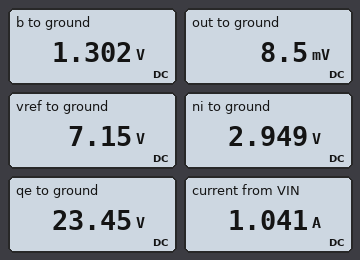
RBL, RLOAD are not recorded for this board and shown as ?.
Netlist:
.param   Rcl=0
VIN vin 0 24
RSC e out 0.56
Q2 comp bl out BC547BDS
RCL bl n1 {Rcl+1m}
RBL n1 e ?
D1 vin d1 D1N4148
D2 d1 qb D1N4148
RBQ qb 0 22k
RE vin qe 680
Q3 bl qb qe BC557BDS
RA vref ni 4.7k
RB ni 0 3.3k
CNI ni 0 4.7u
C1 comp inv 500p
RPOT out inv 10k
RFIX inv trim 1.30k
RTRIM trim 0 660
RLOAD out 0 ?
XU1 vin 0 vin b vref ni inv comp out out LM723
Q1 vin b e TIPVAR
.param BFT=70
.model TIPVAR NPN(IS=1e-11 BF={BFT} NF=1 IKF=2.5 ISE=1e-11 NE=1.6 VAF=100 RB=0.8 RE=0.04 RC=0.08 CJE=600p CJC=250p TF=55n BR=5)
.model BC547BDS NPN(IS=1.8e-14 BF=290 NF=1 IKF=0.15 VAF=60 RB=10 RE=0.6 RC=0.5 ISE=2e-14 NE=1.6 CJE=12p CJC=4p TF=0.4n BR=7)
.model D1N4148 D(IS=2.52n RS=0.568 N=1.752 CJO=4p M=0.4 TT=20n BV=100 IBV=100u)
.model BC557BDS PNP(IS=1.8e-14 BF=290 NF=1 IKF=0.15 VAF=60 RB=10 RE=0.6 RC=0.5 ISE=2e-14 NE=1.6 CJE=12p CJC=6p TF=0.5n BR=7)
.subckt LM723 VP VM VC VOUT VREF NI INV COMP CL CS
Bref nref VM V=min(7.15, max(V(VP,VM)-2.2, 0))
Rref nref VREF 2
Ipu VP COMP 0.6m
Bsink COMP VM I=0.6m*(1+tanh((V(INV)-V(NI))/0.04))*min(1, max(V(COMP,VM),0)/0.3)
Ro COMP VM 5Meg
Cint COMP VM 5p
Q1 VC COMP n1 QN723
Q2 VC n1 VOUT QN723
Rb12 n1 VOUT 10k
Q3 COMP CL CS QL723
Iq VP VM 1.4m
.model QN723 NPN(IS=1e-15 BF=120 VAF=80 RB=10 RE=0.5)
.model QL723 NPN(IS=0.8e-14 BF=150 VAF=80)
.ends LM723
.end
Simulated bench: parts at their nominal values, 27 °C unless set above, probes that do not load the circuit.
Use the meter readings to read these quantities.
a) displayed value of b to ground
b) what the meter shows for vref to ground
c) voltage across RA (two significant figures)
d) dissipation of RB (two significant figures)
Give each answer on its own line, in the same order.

1.302 V
7.15 V
4.2 V
2.6 mW
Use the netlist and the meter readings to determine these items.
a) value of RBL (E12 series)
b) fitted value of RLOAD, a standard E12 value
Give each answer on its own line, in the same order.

56 Ω
8.2 mΩ
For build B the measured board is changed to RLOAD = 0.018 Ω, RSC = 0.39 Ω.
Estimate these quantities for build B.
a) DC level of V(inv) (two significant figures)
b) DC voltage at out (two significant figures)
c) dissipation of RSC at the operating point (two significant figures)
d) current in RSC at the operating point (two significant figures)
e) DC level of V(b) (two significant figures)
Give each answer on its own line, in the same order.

4.4 mV
27 mV
870 mW
1.5 A
1.4 V
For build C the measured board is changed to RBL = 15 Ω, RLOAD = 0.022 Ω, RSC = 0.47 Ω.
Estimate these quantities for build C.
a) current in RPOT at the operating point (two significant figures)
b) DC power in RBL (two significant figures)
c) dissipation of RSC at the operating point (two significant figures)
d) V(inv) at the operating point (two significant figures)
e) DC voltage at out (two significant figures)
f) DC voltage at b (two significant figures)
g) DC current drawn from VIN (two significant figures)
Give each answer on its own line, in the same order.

2.4 µA
9.6 µW
800 mW
4.7 mV
29 mV
1.4 V
1.3 A
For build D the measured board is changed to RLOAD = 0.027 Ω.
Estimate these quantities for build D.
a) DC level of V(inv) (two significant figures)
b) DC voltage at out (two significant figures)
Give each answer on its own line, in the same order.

4.6 mV
28 mV
